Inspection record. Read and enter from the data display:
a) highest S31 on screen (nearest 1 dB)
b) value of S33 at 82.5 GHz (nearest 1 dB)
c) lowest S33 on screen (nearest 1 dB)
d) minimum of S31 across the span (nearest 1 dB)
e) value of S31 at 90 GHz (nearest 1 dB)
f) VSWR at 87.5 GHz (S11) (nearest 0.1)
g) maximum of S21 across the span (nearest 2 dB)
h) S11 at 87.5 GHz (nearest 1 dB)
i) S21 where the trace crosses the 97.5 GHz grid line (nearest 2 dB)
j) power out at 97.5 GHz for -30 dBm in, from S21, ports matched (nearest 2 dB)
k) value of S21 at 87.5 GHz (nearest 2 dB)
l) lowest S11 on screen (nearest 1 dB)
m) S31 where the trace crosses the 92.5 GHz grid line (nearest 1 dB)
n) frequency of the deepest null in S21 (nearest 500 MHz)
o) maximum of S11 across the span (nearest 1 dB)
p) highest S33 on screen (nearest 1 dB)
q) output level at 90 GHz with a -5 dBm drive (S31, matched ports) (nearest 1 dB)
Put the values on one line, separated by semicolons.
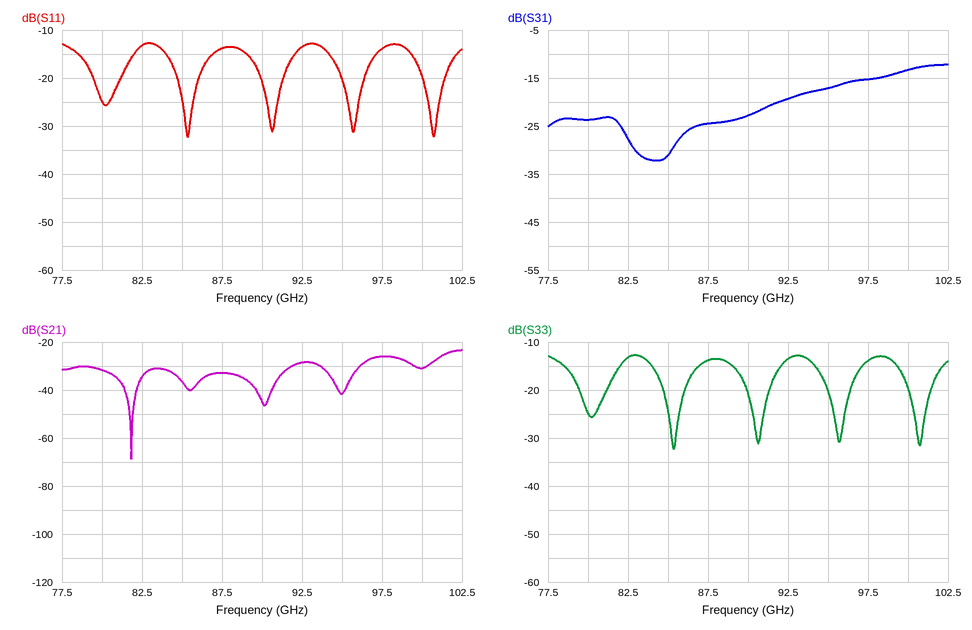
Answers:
-12 dB; -13 dB; -32 dB; -32 dB; -23 dB; 1.5; -24 dB; -14 dB; -26 dB; -56 dBm; -32 dB; -32 dB; -19 dB; 82.0 GHz; -13 dB; -13 dB; -28 dBm
